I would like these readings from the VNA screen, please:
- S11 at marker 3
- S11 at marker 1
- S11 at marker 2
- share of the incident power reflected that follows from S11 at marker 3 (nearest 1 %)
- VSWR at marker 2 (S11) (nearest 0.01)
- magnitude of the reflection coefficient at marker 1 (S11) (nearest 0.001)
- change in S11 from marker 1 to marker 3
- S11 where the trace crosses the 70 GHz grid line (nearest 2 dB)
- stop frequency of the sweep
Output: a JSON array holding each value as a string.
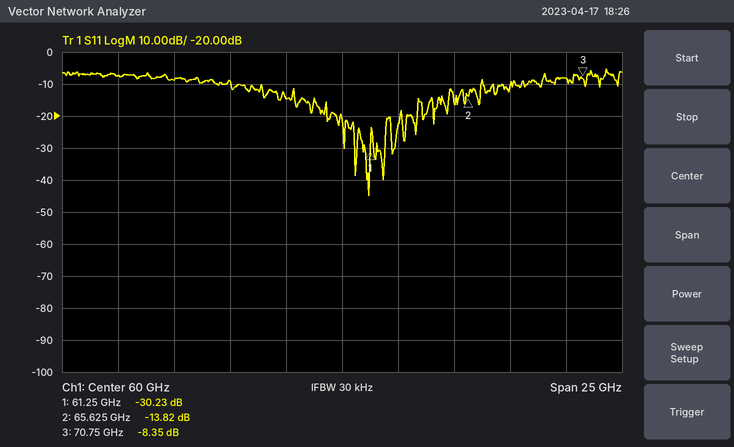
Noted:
["-8.35 dB", "-30.23 dB", "-13.82 dB", "15 %", "1.51", "0.031", "21.88 dB", "-8 dB", "72.5 GHz"]
